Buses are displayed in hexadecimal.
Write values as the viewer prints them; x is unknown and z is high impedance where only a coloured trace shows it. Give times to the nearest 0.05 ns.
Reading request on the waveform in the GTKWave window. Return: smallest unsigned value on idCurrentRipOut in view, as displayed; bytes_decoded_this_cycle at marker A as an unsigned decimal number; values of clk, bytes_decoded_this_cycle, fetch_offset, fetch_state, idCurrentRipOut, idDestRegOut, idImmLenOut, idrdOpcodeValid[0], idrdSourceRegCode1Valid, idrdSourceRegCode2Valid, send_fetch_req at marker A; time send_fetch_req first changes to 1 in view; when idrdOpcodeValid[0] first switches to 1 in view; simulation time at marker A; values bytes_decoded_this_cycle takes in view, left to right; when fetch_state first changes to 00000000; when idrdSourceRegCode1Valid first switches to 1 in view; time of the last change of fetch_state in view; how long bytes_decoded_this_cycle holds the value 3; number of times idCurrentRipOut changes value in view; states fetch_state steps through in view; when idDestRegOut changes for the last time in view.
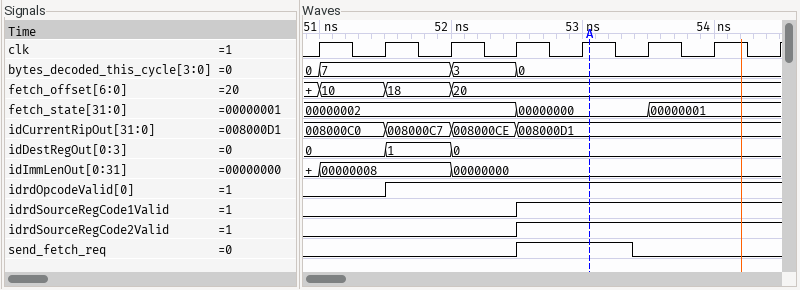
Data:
008000C0
0
clk=1, bytes_decoded_this_cycle=0, fetch_offset=20, fetch_state=00000000, idCurrentRipOut=008000D1, idDestRegOut=0, idImmLenOut=00000000, idrdOpcodeValid[0]=1, idrdSourceRegCode1Valid=1, idrdSourceRegCode2Valid=1, send_fetch_req=1
52.5 ns
51.5 ns
53.05 ns
0, 7, 3, 0
52.5 ns
52.5 ns
53.5 ns
0.5 ns
3
00000002, 00000000, 00000001
52 ns
